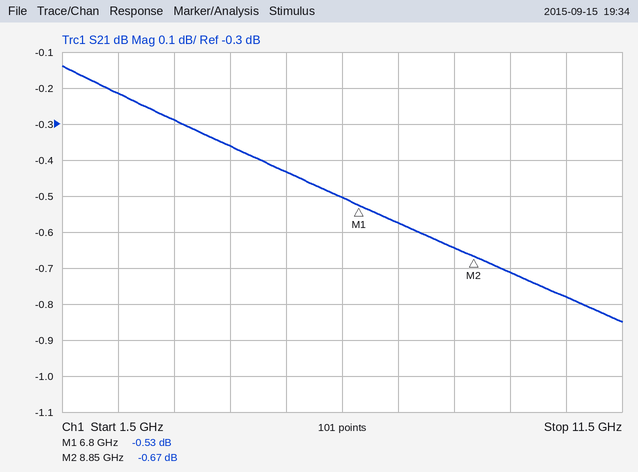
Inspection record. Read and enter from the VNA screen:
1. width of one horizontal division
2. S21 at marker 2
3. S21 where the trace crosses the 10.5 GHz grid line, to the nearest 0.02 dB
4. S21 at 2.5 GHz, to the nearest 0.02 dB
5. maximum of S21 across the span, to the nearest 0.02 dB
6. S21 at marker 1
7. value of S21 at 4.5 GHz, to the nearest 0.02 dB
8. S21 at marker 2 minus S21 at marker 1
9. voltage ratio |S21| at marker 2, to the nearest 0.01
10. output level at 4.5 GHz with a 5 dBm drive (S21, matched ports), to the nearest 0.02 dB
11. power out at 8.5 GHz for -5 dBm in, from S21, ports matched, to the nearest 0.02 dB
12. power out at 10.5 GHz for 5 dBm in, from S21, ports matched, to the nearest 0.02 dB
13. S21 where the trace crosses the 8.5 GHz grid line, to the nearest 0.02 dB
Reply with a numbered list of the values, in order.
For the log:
1. 1 GHz
2. -0.67 dB
3. -0.78 dB
4. -0.22 dB
5. -0.14 dB
6. -0.53 dB
7. -0.36 dB
8. -0.14 dB
9. 0.93
10. 4.64 dBm
11. -5.64 dBm
12. 4.22 dBm
13. -0.64 dB
